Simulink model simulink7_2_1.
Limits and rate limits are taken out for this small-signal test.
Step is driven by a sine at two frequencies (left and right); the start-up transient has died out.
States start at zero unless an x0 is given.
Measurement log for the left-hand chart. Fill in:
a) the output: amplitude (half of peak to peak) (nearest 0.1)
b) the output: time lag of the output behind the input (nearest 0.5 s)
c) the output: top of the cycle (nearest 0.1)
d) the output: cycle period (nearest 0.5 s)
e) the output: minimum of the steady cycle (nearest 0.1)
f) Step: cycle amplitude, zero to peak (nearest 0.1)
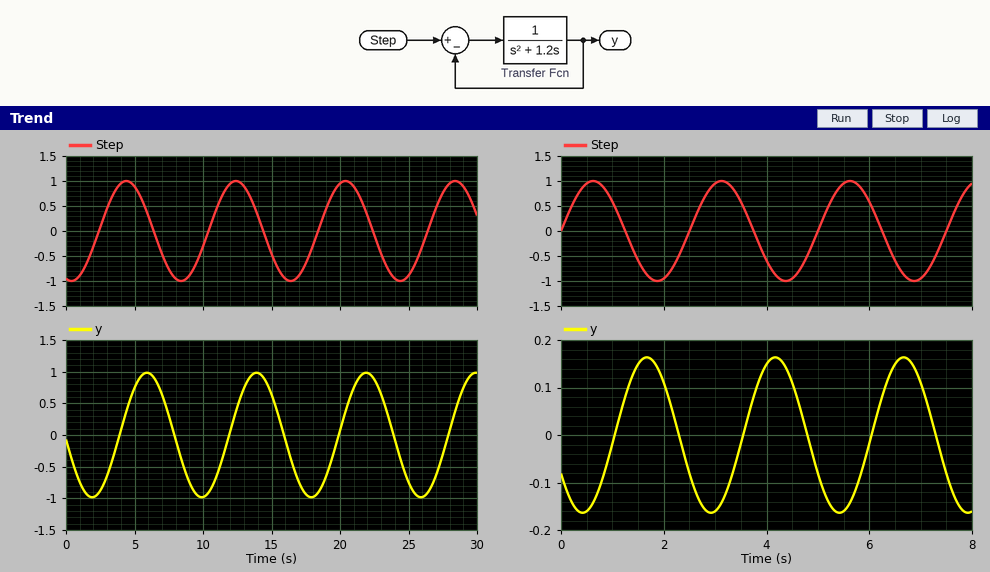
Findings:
1.0
1.5 s
1.0
8.0 s
-1.0
1.0
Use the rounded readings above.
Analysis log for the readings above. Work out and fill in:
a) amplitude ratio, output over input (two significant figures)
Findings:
1.0
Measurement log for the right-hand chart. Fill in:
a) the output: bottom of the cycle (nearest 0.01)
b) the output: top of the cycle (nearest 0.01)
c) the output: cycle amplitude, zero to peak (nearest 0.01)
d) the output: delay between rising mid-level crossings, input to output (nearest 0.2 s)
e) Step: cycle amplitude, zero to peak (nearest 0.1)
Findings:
-0.16
0.16
0.16
1.0 s
1.0
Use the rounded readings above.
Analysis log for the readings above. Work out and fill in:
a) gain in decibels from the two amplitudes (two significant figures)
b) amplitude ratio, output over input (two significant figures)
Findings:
-16 dB
0.16
